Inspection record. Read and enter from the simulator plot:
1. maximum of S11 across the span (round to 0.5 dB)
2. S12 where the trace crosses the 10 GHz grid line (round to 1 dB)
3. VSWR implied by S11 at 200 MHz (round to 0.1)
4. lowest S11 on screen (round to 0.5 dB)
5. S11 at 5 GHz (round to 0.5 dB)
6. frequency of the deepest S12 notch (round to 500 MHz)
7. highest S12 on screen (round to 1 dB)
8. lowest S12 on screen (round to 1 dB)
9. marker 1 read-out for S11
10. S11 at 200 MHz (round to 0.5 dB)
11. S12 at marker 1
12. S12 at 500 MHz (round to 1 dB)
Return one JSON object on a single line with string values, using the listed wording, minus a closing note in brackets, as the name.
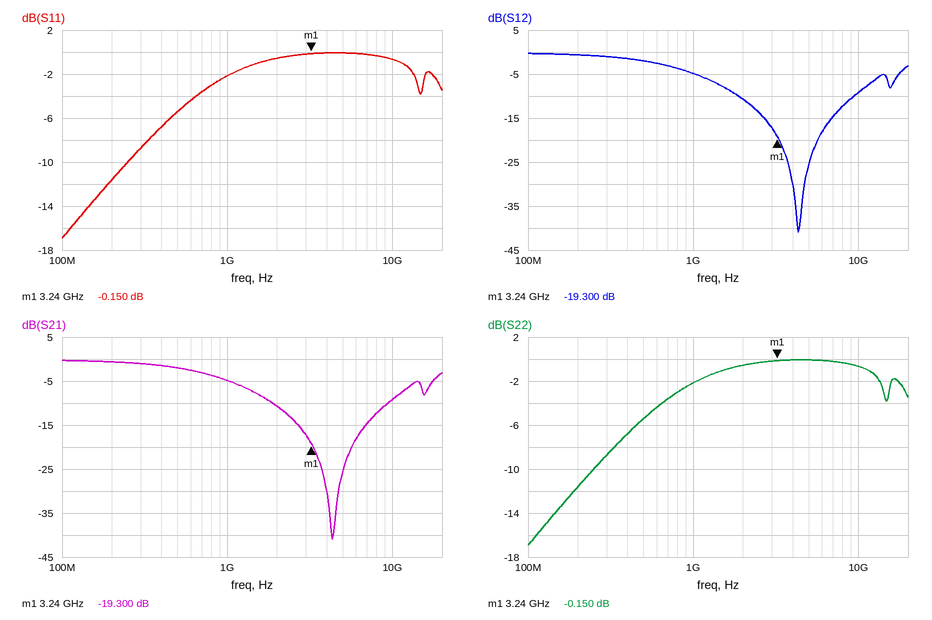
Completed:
{"maximum of S11 across the span": "0.0 dB", "S12 where the trace crosses the 10 GHz grid line": "-9 dB", "VSWR implied by S11 at 200 MHz": "1.7", "lowest S11 on screen": "-17.0 dB", "S11 at 5 GHz": "0.0 dB", "frequency of the deepest S12 notch": "4.5 GHz", "highest S12 on screen": "0 dB", "lowest S12 on screen": "-41 dB", "marker 1 read-out for S11": "-0.150 dB", "S11 at 200 MHz": "-11.5 dB", "S12 at marker 1": "-19.300 dB", "S12 at 500 MHz": "-2 dB"}
